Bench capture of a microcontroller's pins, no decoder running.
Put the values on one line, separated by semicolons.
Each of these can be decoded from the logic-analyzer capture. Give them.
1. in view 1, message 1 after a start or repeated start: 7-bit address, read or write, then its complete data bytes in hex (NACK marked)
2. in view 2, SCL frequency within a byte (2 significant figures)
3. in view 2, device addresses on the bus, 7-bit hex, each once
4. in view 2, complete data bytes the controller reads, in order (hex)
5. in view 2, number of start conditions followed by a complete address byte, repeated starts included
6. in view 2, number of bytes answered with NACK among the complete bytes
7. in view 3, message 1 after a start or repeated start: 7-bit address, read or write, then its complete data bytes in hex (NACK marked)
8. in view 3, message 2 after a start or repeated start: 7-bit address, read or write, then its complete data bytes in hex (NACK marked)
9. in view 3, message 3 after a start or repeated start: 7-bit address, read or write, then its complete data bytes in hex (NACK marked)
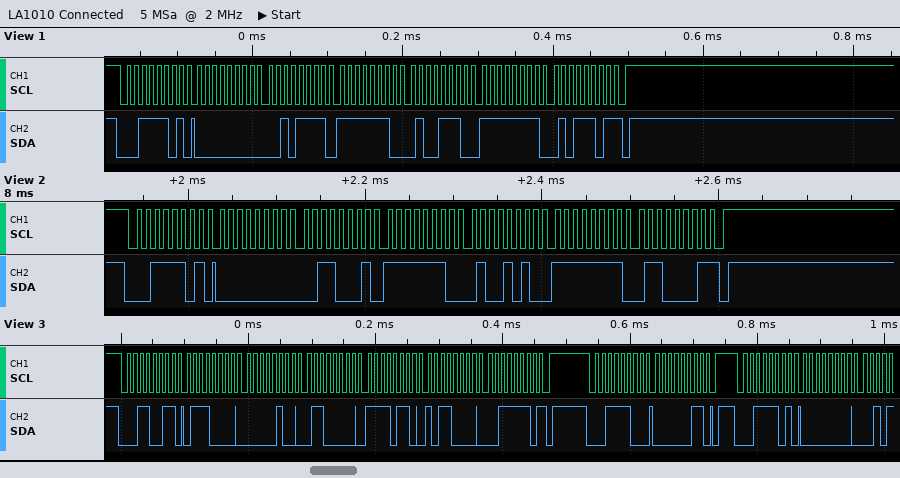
0x1E read: 00 2F FE 4E FF 5D NACK; 100 kHz; 0x1E; 00 31 FE 4A FF 61; 1; 1; 0x19 read: 70 04 60 F6 B0 3E NACK; 0x1E write: 03; 0x1E read: 00
